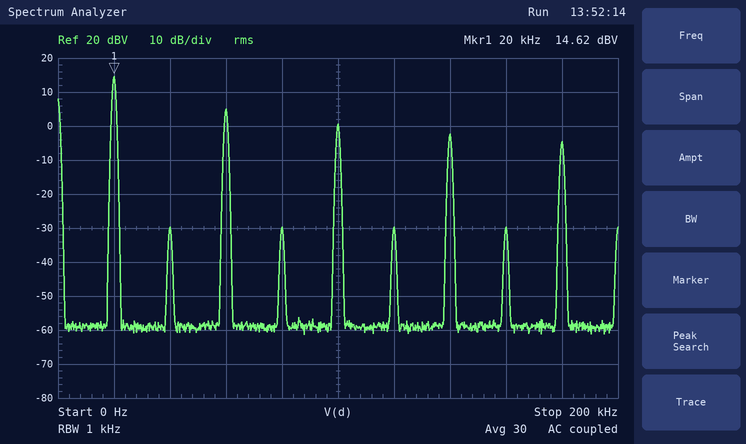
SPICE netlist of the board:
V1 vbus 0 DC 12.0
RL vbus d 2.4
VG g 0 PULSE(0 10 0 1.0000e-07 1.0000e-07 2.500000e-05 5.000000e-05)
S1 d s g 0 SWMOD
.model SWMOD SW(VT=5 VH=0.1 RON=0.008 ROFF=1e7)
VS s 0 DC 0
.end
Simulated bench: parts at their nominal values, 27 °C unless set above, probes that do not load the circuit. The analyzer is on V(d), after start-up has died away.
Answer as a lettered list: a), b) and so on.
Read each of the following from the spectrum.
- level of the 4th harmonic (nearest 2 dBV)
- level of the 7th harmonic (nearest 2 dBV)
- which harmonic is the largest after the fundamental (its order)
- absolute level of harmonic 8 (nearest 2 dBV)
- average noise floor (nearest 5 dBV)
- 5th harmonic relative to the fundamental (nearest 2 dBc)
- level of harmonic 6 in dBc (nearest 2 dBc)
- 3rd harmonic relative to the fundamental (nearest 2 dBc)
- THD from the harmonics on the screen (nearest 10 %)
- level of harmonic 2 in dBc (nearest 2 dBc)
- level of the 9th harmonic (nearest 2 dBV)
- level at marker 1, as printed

a) -30 dBV
b) -2 dBV
c) 3
d) -30 dBV
e) -60 dBV
f) -14 dBc
g) -44 dBc
h) -10 dBc
i) 40 %
j) -44 dBc
k) -4 dBV
l) 14.62 dBV
